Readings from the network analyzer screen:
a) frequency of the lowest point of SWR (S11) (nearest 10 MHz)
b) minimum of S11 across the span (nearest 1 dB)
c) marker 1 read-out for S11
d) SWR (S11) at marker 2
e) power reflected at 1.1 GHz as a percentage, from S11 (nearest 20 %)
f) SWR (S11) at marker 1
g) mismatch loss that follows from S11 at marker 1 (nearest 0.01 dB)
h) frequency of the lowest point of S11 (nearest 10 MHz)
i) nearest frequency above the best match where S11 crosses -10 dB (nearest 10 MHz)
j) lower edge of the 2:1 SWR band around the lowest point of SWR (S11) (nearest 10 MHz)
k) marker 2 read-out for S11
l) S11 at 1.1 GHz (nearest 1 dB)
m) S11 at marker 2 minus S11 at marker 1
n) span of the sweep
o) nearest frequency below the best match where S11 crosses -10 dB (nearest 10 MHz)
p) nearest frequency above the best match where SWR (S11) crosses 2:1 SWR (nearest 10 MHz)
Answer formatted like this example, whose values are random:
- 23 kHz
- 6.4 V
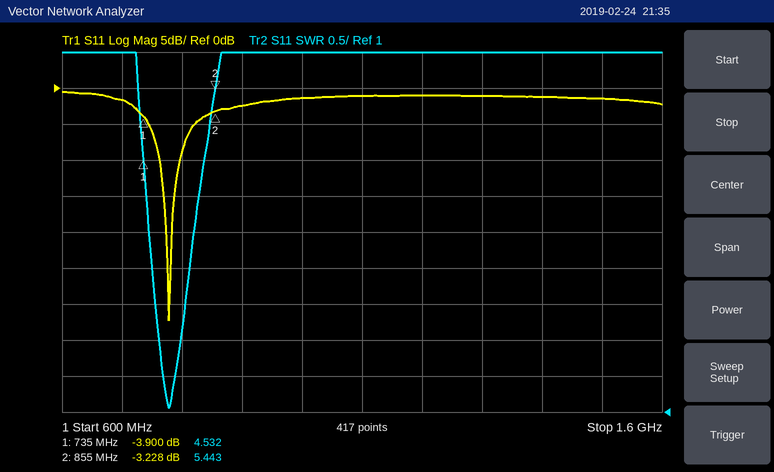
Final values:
- 780 MHz
- -32 dB
- -3.900 dB
- 5.443
- 80 %
- 4.532
- 2.27 dB
- 780 MHz
- 800 MHz
- 760 MHz
- -3.228 dB
- -1 dB
- 0.672 dB
- 1 GHz
- 760 MHz
- 800 MHz
